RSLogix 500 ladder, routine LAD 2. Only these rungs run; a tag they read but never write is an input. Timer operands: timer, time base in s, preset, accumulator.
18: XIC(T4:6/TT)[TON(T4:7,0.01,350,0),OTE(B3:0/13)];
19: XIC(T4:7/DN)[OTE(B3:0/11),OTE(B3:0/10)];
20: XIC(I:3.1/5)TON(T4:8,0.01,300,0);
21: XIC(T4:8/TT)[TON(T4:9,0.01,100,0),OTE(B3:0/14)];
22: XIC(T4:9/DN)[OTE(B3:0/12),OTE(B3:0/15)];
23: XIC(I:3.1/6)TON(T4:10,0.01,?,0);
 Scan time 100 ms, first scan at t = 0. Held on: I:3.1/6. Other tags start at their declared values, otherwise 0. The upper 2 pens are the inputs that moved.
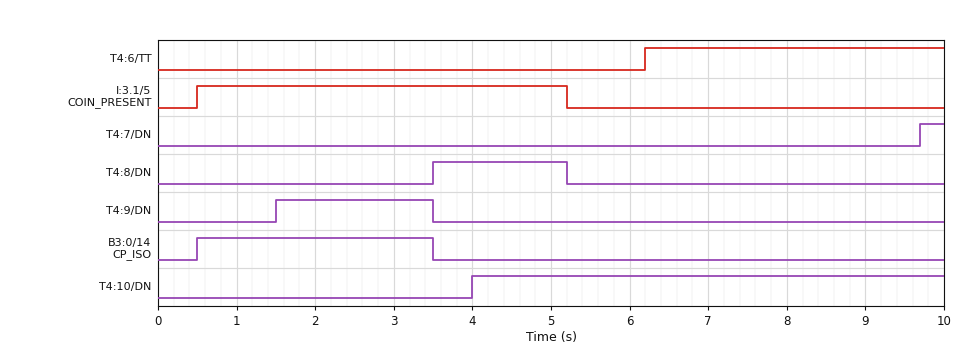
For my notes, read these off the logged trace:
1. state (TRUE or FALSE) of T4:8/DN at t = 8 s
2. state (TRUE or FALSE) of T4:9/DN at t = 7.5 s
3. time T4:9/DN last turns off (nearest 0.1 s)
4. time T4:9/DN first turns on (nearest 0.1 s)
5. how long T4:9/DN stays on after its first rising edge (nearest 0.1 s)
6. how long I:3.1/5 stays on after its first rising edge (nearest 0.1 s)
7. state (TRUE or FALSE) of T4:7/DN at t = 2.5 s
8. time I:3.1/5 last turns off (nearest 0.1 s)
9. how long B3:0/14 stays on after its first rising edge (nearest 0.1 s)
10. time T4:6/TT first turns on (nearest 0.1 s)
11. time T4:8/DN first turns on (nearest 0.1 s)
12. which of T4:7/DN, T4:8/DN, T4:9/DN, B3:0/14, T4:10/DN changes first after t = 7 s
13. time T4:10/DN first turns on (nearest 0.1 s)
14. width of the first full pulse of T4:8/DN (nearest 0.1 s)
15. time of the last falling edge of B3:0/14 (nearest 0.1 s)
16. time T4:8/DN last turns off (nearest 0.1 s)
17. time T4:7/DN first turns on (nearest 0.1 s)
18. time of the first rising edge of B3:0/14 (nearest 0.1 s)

FALSE
FALSE
3.5 s
1.5 s
2.0 s
4.7 s
FALSE
5.2 s
3.0 s
6.2 s
3.5 s
T4:7/DN
4.0 s
1.7 s
3.5 s
5.2 s
9.7 s
0.5 s
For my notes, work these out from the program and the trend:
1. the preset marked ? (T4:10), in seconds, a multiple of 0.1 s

4.0 s
